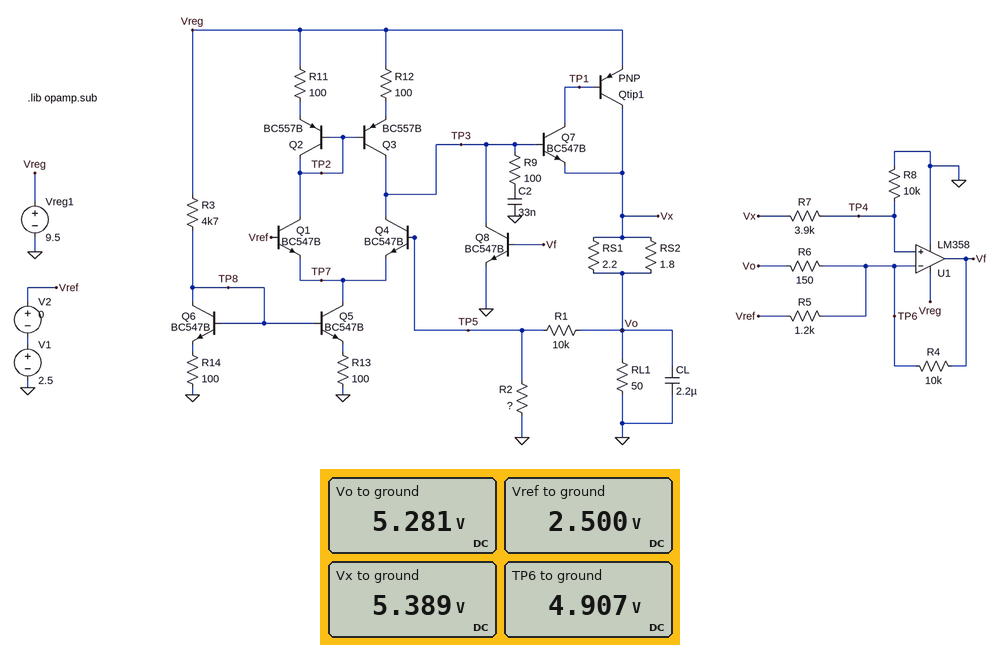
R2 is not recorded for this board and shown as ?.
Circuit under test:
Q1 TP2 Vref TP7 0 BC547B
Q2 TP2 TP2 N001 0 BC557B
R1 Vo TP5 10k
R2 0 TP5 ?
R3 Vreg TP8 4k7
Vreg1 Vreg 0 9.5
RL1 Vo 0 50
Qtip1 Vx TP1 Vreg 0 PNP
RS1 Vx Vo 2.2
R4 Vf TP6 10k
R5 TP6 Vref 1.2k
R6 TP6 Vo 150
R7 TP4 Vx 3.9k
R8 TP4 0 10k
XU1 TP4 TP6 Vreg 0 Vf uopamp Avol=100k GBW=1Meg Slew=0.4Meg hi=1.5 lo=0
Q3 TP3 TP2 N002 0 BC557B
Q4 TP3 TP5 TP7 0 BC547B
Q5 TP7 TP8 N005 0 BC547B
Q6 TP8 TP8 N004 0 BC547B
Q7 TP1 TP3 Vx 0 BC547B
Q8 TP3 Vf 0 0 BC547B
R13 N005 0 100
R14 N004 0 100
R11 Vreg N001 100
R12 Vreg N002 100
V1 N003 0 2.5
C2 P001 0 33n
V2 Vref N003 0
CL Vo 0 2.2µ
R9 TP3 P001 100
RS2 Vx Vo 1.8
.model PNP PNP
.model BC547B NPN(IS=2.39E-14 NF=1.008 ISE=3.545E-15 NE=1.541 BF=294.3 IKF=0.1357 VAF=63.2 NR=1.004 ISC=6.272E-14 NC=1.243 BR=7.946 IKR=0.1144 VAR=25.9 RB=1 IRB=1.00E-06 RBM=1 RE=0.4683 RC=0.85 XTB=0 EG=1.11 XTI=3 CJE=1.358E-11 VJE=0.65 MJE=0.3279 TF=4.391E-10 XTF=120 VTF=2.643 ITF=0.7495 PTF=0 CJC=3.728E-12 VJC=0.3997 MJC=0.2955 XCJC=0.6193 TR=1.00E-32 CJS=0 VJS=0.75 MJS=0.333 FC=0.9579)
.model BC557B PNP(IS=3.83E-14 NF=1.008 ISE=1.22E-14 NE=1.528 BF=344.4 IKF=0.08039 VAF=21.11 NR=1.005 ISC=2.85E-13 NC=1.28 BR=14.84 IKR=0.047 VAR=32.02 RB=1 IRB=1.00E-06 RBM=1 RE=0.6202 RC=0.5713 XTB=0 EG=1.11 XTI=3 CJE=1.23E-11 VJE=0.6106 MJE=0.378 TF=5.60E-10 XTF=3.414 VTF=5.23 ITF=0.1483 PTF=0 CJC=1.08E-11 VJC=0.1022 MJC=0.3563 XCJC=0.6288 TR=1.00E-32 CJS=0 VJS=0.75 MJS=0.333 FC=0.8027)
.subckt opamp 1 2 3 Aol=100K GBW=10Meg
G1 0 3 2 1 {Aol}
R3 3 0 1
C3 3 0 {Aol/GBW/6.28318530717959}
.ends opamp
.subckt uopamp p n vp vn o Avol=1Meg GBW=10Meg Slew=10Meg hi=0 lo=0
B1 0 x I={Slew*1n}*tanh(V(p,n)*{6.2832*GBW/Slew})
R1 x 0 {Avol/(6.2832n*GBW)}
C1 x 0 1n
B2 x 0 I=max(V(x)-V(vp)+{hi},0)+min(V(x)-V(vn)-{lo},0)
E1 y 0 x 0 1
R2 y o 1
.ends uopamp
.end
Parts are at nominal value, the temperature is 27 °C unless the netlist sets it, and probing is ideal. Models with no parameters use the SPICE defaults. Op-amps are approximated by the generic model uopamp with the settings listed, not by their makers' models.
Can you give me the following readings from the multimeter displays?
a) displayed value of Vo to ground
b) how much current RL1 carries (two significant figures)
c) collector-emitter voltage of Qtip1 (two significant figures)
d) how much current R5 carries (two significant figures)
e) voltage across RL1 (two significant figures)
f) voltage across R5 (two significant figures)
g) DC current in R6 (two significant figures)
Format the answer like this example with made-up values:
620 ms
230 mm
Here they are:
5.281 V
110 mA
-4.1 V
2.0 mA
5.3 V
2.4 V
2.5 mA
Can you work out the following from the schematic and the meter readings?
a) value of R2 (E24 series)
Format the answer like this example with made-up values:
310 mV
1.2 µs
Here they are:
9.1 kΩ
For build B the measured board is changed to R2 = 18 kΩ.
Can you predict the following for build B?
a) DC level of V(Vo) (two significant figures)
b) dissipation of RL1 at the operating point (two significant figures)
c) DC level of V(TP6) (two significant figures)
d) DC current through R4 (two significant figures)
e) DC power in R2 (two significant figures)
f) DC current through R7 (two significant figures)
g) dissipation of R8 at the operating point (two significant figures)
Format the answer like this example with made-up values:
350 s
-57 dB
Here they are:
3.9 V
310 mW
3.7 V
370 µA
350 µW
290 µA
830 µW
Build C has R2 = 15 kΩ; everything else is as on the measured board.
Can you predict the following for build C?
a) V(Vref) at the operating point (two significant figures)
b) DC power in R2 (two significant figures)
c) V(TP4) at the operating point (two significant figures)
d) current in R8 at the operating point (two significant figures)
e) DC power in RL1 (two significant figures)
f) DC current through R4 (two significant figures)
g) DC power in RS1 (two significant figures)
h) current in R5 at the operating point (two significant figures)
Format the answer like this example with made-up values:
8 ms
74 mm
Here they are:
2.5 V
420 µW
3.1 V
310 µA
350 mW
400 µA
3.3 mW
1.2 mA
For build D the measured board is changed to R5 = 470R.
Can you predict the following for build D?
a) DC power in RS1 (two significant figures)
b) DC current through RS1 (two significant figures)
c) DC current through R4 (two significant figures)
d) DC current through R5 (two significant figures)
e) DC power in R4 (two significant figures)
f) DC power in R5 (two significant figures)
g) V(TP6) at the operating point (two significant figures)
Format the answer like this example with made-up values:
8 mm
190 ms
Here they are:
5.5 mW
50 mA
460 µA
4.4 mA
2.1 mW
9.0 mW
4.6 V
